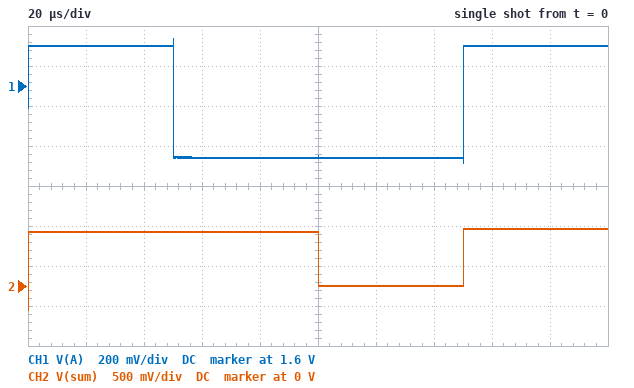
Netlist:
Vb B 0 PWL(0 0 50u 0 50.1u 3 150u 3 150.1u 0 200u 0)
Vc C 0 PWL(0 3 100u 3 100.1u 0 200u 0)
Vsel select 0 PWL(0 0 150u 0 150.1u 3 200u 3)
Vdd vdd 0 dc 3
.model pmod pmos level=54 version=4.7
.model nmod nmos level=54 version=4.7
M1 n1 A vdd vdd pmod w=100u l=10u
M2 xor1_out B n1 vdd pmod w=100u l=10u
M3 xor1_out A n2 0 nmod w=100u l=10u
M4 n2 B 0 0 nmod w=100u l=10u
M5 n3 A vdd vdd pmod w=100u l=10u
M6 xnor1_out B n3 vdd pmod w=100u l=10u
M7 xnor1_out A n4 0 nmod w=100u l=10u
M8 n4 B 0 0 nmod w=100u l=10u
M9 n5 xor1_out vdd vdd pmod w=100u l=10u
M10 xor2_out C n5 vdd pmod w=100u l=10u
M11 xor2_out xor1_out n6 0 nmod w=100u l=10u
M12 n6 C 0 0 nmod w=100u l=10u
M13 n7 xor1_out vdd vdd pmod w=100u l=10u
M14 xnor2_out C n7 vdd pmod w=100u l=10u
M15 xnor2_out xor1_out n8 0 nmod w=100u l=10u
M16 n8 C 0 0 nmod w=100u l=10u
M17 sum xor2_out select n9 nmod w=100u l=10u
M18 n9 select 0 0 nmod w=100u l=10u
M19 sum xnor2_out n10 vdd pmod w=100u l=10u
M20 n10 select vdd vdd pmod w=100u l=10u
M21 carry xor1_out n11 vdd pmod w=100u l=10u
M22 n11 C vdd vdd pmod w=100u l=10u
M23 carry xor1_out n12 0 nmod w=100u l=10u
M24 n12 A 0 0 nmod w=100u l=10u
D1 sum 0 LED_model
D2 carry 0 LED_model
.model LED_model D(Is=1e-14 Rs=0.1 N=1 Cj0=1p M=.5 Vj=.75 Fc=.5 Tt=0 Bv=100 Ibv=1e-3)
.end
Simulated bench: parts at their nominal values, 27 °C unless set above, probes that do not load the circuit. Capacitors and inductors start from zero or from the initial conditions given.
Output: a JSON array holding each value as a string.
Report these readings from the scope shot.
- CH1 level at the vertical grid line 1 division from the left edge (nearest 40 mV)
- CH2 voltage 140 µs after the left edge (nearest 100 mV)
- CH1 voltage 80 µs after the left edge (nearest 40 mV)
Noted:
["1.80 V", "0 V", "1.24 V"]
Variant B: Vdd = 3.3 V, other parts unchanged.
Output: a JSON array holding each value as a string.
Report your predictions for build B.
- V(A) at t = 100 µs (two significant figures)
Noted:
["1.4 V"]
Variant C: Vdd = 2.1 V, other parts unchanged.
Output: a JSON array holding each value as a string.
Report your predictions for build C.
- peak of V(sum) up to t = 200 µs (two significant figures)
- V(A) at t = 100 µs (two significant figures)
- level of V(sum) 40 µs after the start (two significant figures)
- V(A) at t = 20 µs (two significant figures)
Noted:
["690 mV", "880 mV", "660 mV", "1.2 V"]
